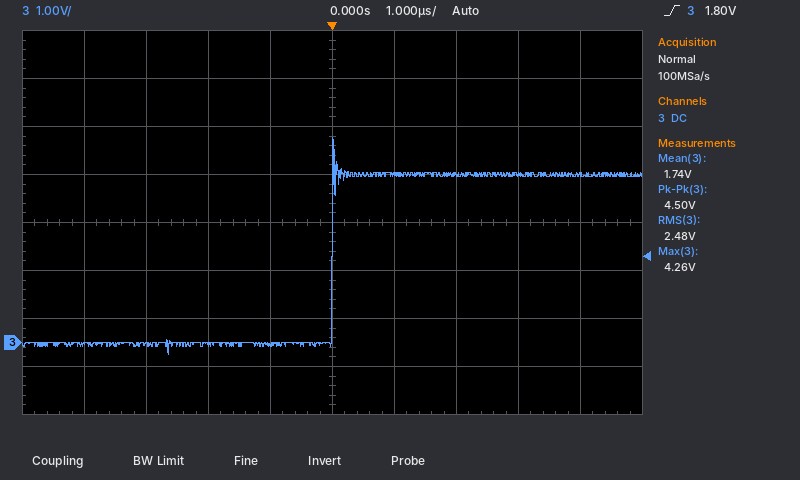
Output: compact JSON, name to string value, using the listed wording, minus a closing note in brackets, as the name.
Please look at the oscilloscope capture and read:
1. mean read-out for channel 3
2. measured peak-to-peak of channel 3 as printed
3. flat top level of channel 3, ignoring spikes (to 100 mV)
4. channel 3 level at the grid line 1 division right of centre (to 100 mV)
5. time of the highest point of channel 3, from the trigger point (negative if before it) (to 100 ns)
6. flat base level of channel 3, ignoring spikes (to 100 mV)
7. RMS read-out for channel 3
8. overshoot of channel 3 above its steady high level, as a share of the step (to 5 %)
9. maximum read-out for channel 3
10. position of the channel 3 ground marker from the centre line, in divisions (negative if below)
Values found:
{"mean read-out for channel 3": "1.74 V", "measured peak-to-peak of channel 3 as printed": "4.50 V", "flat top level of channel 3, ignoring spikes": "3.5 V", "channel 3 level at the grid line 1 division right of centre": "3.5 V", "time of the highest point of channel 3, from the trigger point (negative if before it)": "0.0 µs", "flat base level of channel 3, ignoring spikes": "0.0 V", "RMS read-out for channel 3": "2.48 V", "overshoot of channel 3 above its steady high level, as a share of the step": "20 %", "maximum read-out for channel 3": "4.26 V", "position of the channel 3 ground marker from the centre line, in divisions": "-2.5 div"}
